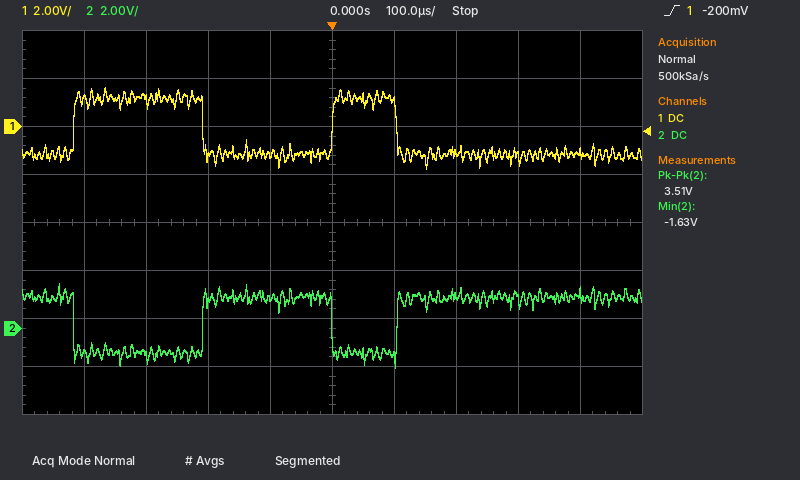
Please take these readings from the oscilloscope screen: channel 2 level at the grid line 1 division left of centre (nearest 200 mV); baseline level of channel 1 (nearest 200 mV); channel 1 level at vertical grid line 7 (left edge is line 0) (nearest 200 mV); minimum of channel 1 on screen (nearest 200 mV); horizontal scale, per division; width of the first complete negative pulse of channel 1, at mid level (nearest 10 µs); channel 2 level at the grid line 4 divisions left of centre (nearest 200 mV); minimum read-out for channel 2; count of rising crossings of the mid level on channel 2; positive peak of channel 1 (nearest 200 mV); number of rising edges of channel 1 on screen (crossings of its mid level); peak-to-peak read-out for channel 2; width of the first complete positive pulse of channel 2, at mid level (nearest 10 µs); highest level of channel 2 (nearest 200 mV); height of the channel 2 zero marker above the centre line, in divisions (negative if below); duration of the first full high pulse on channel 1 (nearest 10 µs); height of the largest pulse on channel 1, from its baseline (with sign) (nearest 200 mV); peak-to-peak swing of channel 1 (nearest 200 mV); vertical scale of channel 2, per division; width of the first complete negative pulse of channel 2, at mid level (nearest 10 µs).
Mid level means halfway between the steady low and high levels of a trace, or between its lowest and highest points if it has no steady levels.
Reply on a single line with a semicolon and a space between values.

1.2 V; -1.2 V; -1.2 V; -1.8 V; 100 µs; 210 µs; -1.0 V; -1.63 V; 2; 1.6 V; 2; 3.51 V; 210 µs; 1.8 V; -2.2 div; 210 µs; +2.8 V; 3.4 V; 2 V; 210 µs
